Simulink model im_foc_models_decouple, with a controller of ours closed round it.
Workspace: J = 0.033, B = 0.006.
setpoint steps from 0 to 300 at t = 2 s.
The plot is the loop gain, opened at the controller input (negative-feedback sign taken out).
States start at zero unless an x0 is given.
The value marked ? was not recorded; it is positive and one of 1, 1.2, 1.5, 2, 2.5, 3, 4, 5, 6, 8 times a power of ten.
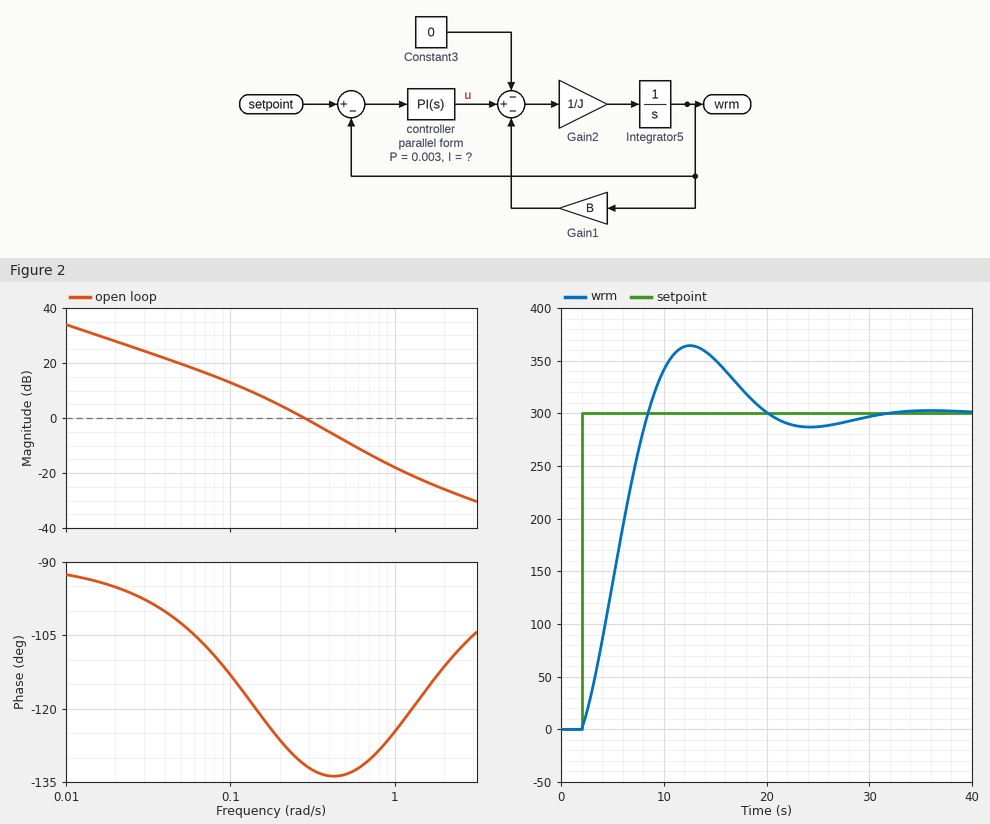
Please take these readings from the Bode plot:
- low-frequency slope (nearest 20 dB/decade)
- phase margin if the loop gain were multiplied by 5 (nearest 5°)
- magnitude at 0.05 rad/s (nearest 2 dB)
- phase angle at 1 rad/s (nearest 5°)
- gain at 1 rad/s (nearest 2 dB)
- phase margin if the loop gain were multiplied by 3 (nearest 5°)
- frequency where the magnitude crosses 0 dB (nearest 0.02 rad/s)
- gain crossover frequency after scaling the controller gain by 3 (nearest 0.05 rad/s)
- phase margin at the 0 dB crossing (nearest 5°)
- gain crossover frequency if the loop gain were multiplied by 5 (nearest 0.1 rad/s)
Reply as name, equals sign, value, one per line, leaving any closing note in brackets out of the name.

low-frequency slope = -20 dB/decade
phase margin if the loop gain were multiplied by 5 = 50°
magnitude at 0.05 rad/s = 20 dB
phase angle at 1 rad/s = -125°
gain at 1 rad/s = -18 dB
phase margin if the loop gain were multiplied by 3 = 45°
frequency where the magnitude crosses 0 dB = 0.28 rad/s
gain crossover frequency after scaling the controller gain by 3 = 0.55 rad/s
phase margin at the 0 dB crossing = 50°
gain crossover frequency if the loop gain were multiplied by 5 = 0.7 rad/s
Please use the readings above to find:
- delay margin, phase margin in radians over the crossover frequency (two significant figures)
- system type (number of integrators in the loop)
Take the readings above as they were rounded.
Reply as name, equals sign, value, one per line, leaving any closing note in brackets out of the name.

delay margin, phase margin in radians over the crossover frequency = 3.1 s
system type = 1
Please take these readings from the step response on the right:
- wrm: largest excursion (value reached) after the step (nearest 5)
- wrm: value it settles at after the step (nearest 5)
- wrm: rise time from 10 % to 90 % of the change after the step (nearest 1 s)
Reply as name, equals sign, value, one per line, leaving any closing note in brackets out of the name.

wrm: largest excursion (value reached) after the step = 365
wrm: value it settles at after the step = 300
wrm: rise time from 10 % to 90 % of the change after the step = 5 s
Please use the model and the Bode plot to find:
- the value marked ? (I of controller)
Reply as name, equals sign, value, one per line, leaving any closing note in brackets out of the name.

the value marked ? = 0.003
